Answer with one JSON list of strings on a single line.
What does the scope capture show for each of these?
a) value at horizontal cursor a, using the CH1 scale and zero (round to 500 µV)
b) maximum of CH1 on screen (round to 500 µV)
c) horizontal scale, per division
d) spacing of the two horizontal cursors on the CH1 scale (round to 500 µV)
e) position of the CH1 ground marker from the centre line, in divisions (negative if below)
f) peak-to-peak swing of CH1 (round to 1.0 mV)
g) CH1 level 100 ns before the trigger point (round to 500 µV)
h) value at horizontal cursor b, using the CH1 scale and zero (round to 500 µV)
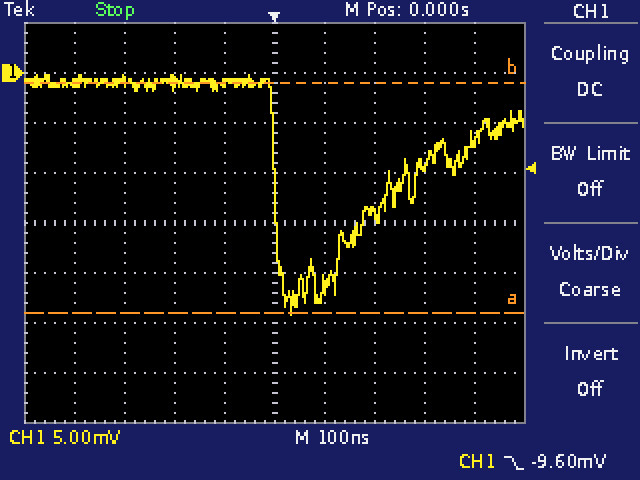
["-24.0 mV", "0.0 mV", "100 ns", "23.0 mV", "+3.0 div", "24.0 mV", "-1.0 mV", "-1.0 mV"]
